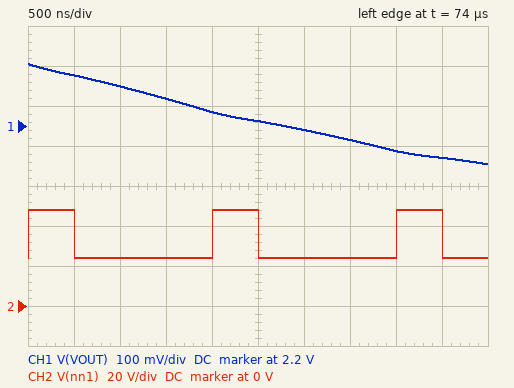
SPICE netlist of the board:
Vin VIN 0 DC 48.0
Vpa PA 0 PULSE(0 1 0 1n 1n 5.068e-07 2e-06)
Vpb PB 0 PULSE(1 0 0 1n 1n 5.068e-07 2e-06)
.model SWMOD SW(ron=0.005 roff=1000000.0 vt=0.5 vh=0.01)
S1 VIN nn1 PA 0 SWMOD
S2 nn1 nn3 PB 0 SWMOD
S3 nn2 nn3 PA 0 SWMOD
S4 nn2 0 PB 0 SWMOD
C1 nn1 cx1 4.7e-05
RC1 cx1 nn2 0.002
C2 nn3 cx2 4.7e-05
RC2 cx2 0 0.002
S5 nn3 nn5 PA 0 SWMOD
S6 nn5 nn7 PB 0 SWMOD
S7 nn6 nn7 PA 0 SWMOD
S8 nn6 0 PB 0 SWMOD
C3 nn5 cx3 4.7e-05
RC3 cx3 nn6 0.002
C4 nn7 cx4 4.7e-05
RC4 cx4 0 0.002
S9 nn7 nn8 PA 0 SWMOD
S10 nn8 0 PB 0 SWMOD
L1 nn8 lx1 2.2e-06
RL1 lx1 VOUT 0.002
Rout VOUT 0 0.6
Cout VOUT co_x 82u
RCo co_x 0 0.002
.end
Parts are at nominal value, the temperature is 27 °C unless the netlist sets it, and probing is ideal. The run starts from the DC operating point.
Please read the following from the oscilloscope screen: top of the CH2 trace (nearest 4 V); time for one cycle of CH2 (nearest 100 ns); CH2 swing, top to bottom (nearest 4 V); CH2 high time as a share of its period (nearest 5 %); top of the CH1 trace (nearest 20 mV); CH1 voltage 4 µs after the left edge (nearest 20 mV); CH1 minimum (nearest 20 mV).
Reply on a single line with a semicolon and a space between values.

48 V; 2.0 µs; 24 V; 25 %; 2.36 V; 2.14 V; 2.10 V
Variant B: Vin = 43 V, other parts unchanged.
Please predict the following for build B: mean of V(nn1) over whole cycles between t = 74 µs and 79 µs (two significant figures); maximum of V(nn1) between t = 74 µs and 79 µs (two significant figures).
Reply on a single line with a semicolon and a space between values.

27 V; 43 V
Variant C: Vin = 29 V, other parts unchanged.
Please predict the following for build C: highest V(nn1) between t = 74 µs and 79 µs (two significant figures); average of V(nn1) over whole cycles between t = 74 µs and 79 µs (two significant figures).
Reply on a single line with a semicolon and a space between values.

29 V; 18 V
